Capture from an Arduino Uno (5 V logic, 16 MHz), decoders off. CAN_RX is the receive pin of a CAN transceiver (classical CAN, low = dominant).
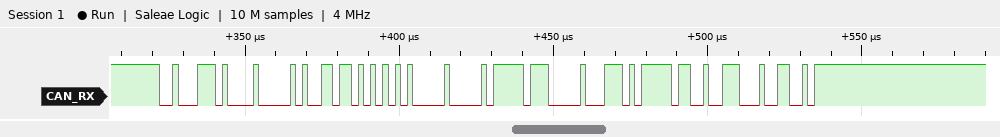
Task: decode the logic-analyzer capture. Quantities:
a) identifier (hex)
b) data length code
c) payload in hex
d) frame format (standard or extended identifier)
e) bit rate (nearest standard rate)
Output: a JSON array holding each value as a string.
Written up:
["0x23A", "8", "13 6A A8 00 FF 00 EB F9", "standard", "500 kbit/s"]
